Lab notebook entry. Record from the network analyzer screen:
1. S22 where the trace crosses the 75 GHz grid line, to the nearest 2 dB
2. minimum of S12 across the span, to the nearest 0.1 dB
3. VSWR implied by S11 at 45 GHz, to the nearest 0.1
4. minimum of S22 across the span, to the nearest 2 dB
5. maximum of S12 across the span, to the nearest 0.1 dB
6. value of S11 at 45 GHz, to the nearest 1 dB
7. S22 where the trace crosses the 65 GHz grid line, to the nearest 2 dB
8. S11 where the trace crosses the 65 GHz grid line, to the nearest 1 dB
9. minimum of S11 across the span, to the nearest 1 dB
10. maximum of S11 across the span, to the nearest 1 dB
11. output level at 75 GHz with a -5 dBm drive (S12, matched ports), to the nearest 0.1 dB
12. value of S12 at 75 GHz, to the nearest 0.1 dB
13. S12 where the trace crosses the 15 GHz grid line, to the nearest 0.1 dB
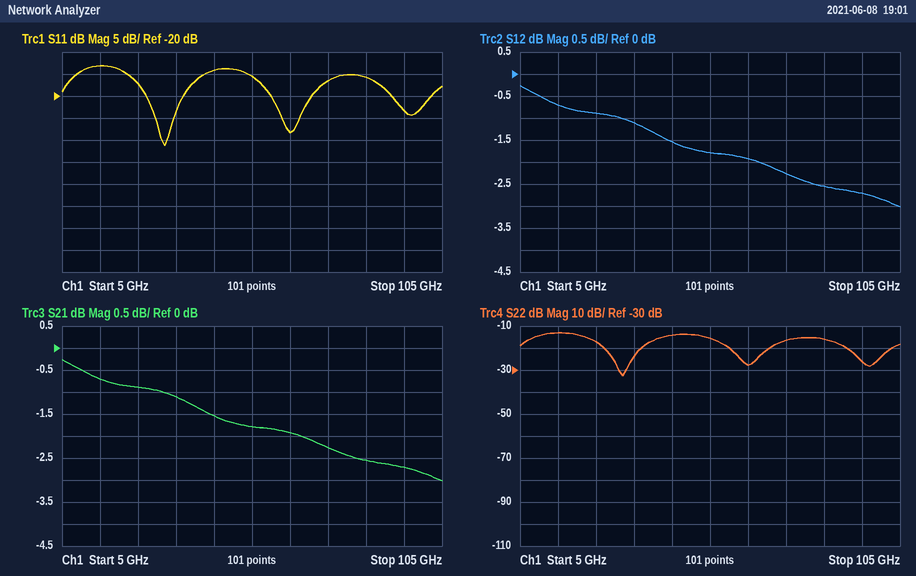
-16 dB
-3.0 dB
1.5
-32 dB
-0.3 dB
-14 dB
-28 dB
-28 dB
-31 dB
-13 dB
-7.3 dBm
-2.3 dB
-0.7 dB
